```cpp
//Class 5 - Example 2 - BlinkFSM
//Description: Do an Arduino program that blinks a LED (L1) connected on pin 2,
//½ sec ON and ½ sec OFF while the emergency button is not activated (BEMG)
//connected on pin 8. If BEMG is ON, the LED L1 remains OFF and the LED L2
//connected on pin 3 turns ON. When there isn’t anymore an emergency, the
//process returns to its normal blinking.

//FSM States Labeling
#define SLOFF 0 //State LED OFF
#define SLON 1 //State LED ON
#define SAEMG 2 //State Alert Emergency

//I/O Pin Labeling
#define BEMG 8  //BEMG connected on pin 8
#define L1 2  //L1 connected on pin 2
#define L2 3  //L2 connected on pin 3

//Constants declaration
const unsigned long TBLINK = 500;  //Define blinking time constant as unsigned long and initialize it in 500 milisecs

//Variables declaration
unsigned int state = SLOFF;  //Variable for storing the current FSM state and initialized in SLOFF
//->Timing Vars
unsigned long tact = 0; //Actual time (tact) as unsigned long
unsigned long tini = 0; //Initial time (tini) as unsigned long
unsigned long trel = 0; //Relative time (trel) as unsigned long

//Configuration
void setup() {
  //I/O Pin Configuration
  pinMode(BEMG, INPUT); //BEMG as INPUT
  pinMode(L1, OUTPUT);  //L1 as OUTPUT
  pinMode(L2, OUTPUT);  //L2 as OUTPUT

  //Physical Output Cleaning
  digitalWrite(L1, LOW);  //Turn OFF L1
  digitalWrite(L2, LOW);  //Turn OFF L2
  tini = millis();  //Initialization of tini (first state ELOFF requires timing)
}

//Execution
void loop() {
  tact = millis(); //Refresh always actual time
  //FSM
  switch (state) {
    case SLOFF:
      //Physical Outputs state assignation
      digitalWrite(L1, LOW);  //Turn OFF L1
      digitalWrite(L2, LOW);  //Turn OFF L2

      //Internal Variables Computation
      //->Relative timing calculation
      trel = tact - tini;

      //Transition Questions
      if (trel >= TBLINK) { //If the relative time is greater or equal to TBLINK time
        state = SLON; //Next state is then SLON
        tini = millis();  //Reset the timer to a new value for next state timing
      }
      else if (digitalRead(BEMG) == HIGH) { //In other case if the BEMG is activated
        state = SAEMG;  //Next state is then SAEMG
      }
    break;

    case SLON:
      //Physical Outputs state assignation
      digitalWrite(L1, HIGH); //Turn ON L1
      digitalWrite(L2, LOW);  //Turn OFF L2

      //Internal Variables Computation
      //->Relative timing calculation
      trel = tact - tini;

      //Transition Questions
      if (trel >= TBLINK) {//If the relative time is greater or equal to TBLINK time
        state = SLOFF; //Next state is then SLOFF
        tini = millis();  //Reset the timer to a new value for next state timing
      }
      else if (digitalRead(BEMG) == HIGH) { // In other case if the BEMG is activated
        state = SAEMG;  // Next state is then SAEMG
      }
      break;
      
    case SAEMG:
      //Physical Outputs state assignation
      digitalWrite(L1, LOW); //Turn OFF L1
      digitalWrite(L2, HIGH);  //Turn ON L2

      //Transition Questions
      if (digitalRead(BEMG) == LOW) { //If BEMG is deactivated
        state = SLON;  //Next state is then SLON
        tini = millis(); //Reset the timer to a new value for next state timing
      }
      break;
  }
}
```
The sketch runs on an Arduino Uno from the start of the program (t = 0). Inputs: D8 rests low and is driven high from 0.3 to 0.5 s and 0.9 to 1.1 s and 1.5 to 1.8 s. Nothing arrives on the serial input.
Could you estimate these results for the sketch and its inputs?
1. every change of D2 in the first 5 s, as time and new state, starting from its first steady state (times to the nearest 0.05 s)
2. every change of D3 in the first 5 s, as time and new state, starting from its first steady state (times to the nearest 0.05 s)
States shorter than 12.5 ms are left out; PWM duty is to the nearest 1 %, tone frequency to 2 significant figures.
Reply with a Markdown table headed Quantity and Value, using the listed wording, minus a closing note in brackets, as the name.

| Quantity | Value |
|---|---|
| every change of D2 in the first 5 s, as time and new state, starting from its first steady state | 0 s low; 0.5 s high; 0.9 s low; 1.1 s high; 1.5 s low; 1.8 s high; 2.3 s low; 2.8 s high; 3.3 s low; 3.8 s high; 4.3 s low; 4.8 s high |
| every change of D3 in the first 5 s, as time and new state, starting from its first steady state | 0 s low; 0.3 s high; 0.5 s low; 0.9 s high; 1.1 s low; 1.5 s high; 1.8 s low |
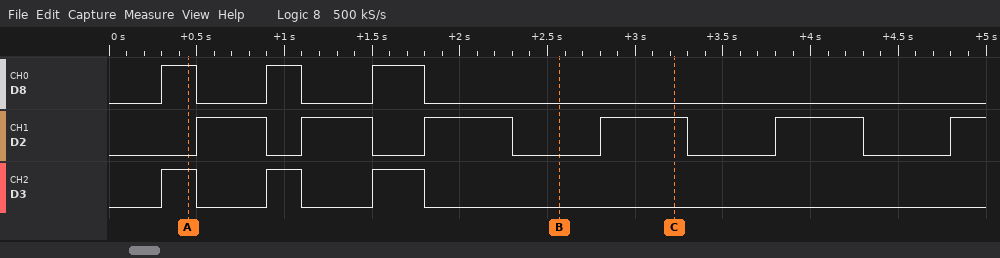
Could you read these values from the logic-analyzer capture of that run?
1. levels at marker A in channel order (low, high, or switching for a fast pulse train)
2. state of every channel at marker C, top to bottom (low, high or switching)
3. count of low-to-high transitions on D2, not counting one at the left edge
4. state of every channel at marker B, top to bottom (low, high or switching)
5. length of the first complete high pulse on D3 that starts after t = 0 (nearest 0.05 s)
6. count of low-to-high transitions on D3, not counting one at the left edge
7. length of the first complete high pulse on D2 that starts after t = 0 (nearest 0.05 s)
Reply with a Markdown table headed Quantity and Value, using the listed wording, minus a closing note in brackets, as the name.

| Quantity | Value |
|---|---|
| levels at marker A in channel order | D8 high, D2 low, D3 high |
| state of every channel at marker C, top to bottom | D8 low, D2 high, D3 low |
| count of low-to-high transitions on D2, not counting one at the left edge | 6 |
| state of every channel at marker B, top to bottom | D8 low, D2 low, D3 low |
| length of the first complete high pulse on D3 that starts after t = 0 | 0.20 s |
| count of low-to-high transitions on D3, not counting one at the left edge | 3 |
| length of the first complete high pulse on D2 that starts after t = 0 | 0.40 s |
